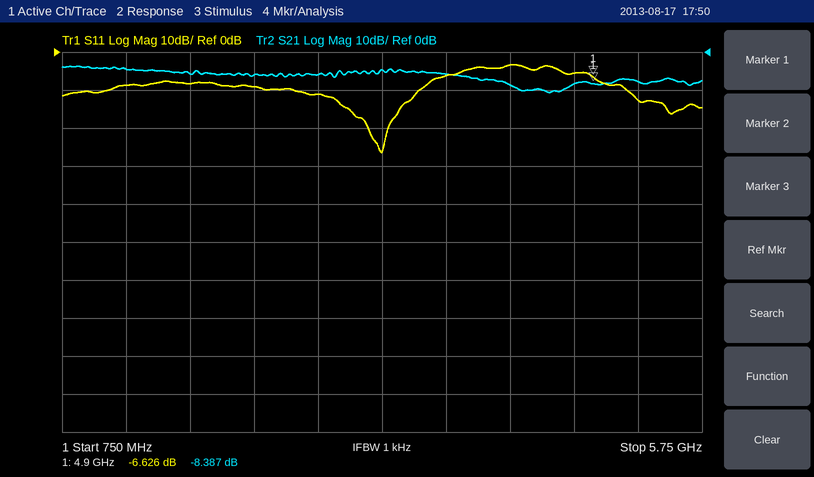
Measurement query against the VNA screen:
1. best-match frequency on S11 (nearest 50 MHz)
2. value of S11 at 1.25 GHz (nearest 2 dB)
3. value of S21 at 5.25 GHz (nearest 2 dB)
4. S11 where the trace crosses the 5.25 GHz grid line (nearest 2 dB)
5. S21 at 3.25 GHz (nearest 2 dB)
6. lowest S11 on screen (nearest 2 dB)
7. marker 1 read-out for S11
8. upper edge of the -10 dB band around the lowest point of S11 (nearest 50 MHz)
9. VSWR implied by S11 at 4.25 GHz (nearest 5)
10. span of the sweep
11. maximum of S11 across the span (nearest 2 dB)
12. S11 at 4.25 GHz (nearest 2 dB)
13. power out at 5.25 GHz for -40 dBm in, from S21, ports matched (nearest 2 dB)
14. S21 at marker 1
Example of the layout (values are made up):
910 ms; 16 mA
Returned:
3.25 GHz; -8 dB; -8 dB; -12 dB; -4 dB; -26 dB; -6.626 dB; 3.55 GHz; 5; 5 GHz; -4 dB; -4 dB; -48 dBm; -8.387 dB
